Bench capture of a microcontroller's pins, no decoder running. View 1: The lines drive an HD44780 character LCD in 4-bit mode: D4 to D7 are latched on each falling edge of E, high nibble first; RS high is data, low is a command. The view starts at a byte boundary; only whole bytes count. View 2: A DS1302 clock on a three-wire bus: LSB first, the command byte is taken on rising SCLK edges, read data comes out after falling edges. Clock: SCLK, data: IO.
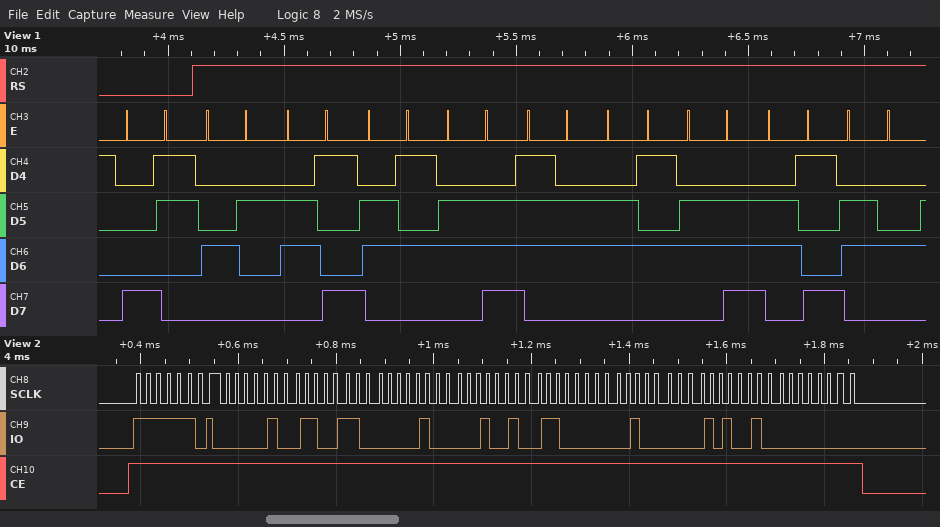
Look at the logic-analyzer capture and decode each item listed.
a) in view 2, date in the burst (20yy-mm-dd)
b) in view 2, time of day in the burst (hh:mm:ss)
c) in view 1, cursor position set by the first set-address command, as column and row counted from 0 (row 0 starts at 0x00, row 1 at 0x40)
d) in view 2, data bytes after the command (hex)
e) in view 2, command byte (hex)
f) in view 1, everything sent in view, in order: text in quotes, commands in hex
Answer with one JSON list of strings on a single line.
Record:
["2025-03-24", "10:33:20", "column 3, row 0", "20 33 10 24 03 02 25 00", "0xBF", "0x83 \"Bienvenid\""]
